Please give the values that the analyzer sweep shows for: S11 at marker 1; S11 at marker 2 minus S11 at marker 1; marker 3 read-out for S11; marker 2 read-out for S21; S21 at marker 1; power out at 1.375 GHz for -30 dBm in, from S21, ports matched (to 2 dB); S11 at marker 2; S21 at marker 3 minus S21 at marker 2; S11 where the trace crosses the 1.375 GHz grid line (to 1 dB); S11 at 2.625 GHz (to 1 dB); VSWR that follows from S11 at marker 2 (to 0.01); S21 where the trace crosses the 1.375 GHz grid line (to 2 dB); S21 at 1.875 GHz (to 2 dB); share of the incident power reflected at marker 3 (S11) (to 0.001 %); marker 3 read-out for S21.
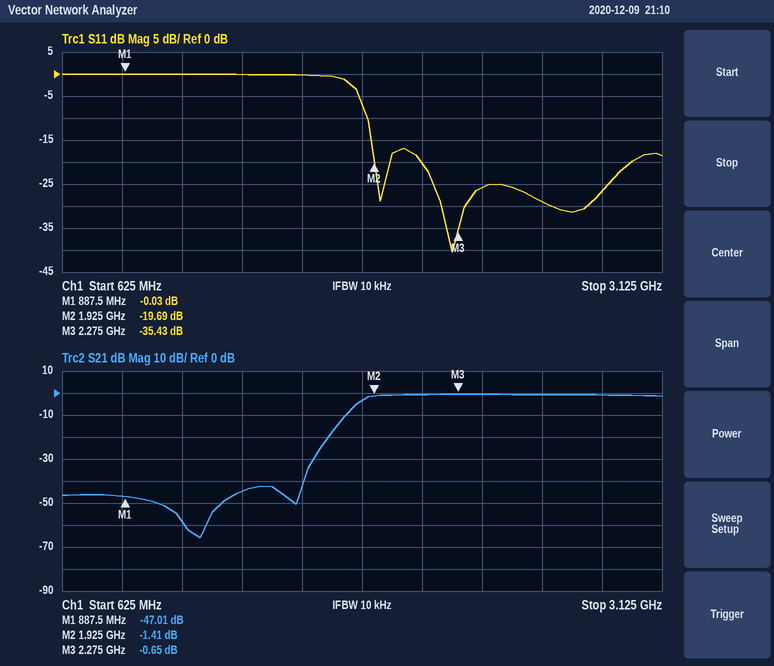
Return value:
-0.03 dB
-19.66 dB
-35.43 dB
-1.41 dB
-47.01 dB
-74 dBm
-19.69 dB
0.76 dB
0 dB
-29 dB
1.23
-44 dB
-4 dB
0.029 %
-0.65 dB
